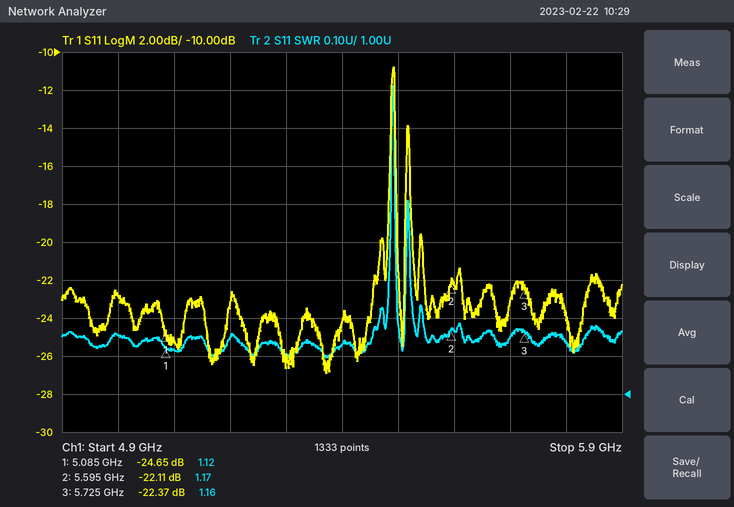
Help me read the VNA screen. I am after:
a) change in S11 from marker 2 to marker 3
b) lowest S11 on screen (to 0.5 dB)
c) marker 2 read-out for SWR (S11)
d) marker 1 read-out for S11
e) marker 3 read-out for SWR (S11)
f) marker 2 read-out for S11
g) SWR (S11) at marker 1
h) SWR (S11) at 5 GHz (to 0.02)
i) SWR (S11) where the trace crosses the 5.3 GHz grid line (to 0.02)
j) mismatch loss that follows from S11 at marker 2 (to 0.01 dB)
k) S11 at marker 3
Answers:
-0.26 dB
-27.0 dB
1.17
-24.65 dB
1.16
-22.11 dB
1.12
1.16
1.10
0.03 dB
-22.37 dB
